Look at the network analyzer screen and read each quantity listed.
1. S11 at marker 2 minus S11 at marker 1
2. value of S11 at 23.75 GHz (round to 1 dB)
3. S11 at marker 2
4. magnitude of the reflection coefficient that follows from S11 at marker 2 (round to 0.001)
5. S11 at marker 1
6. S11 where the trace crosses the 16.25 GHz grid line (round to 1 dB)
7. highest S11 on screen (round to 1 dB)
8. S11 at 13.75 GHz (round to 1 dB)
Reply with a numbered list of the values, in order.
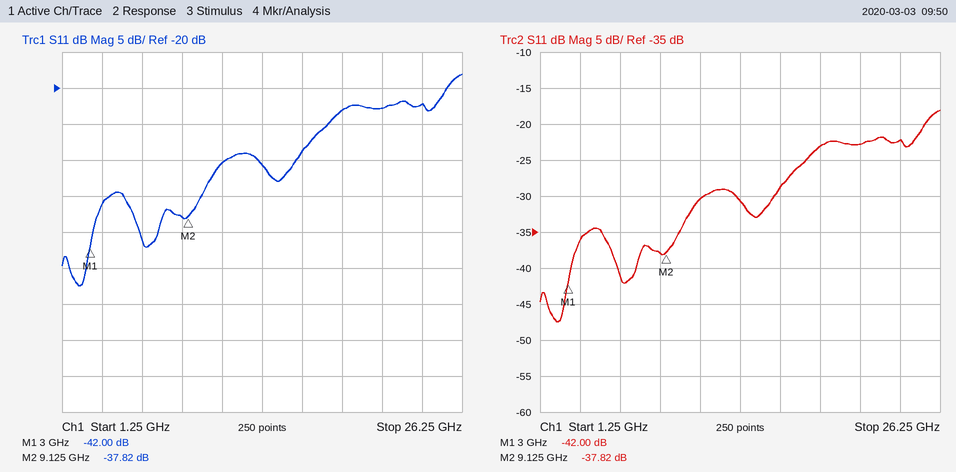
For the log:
1. 4.18 dB
2. -22 dB
3. -37.82 dB
4. 0.013
5. -42.00 dB
6. -29 dB
7. -18 dB
8. -31 dB
